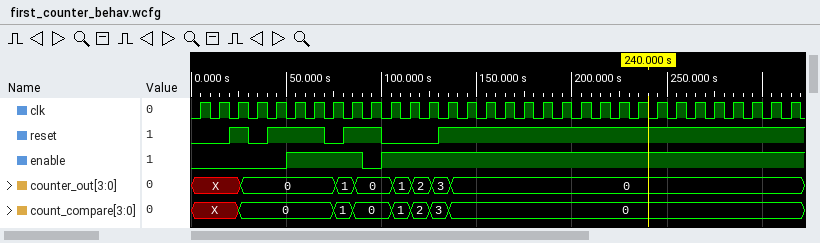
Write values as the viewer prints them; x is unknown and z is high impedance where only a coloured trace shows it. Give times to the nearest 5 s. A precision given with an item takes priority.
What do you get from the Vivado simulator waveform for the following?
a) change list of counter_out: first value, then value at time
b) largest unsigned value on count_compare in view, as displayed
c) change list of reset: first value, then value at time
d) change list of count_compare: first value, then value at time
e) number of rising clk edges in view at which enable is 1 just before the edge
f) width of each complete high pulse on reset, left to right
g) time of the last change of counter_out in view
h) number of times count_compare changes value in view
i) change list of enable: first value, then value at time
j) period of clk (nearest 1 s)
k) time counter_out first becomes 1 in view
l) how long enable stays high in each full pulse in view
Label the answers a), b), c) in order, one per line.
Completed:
a) X, 0 at 25 s, 1 at 75 s, 0 at 85 s, 1 at 105 s, 2 at 115 s, 3 at 125 s, 0 at 135 s
b) 3
c) 0, 1 at 20 s, 0 at 30 s, 1 at 40 s, 0 at 70 s, 1 at 80 s, 0 at 100 s, 1 at 130 s
d) X, 0 at 25 s, 1 at 75 s, 0 at 85 s, 1 at 105 s, 2 at 115 s, 3 at 125 s, 0 at 135 s
e) 26
f) 10 s, 30 s, 20 s
g) 135 s
h) 7
i) 0, 1 at 50 s, 0 at 90 s, 1 at 100 s
j) 10 s
k) 75 s
l) 40 s
